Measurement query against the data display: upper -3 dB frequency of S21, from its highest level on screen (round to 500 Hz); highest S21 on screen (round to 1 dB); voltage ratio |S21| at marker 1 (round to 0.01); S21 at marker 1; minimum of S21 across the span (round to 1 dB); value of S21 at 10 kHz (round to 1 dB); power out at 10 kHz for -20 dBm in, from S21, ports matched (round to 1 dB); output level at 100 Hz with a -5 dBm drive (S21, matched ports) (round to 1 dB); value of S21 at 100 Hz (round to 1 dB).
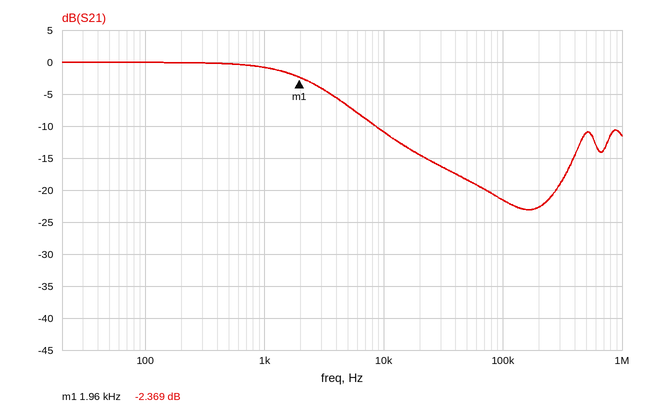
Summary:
2.5 kHz
0 dB
0.76
-2.369 dB
-23 dB
-11 dB
-31 dBm
-5 dBm
0 dB
